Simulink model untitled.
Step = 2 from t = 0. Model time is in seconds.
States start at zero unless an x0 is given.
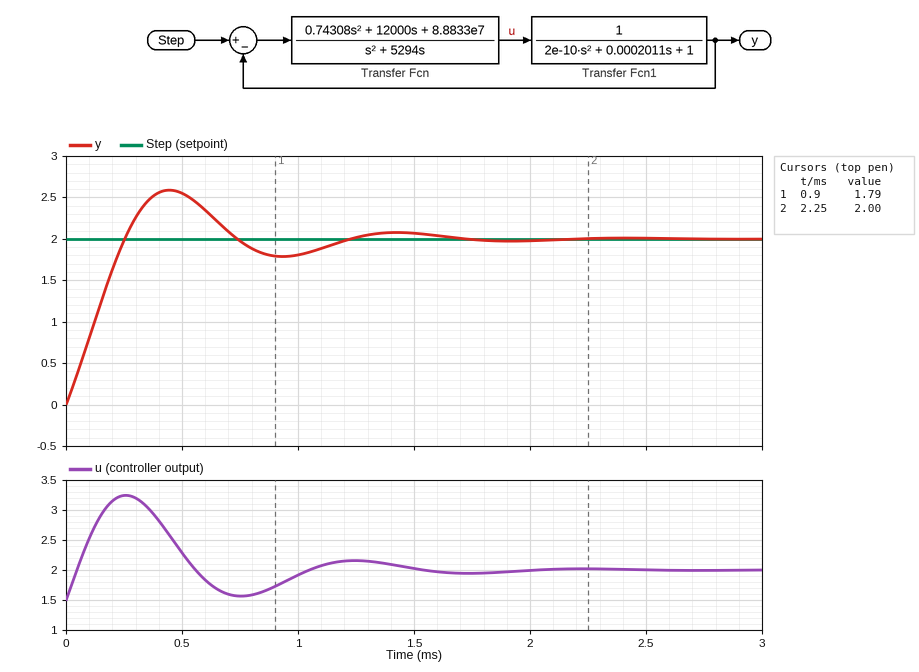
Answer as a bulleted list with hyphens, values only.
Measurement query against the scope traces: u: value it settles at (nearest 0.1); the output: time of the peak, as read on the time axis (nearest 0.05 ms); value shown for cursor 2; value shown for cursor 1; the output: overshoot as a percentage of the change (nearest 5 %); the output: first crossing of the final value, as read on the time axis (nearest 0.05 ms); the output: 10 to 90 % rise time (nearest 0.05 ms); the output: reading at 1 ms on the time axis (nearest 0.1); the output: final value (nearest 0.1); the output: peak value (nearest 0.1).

- 2.0
- 0.45 ms
- 2.00
- 1.79
- 30 %
- 0.25 ms
- 0.20 ms
- 1.8
- 2.0
- 2.6
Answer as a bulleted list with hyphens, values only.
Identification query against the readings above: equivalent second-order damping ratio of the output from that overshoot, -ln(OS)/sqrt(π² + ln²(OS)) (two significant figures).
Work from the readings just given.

- 0.36
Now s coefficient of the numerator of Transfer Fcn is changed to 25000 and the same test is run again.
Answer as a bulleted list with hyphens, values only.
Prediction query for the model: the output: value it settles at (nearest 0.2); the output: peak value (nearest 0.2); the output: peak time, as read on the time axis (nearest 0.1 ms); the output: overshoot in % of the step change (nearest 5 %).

- 2.0
- 2.4
- 0.3 ms
- 20 %
